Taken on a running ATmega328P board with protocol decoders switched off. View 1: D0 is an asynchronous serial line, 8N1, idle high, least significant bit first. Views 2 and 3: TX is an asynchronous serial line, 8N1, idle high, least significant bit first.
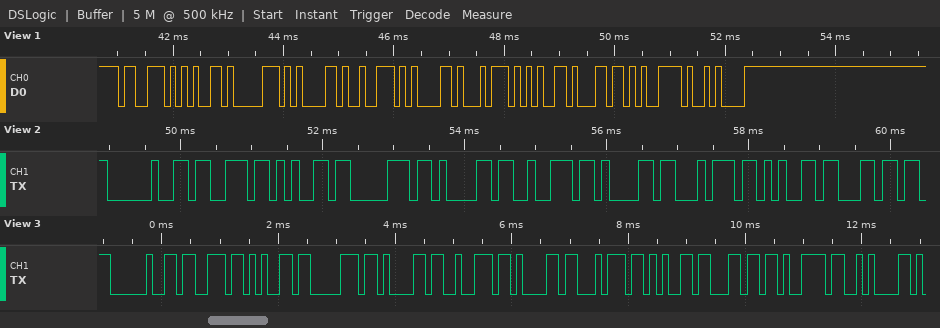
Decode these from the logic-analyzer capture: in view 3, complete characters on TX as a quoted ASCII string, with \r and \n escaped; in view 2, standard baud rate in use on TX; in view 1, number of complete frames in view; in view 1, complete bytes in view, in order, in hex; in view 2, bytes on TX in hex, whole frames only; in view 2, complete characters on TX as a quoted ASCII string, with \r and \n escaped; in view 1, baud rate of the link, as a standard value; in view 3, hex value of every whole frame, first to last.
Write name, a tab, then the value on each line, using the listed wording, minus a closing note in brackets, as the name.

in view 3, complete characters on TX as a quoted ASCII string, with \r and \n escaped	" separately\n"
in view 2, standard baud rate in use on TX	9600 baud
in view 1, number of complete frames in view	11
in view 1, complete bytes in view, in order, in hex	73 65 70 61 72 61 74 65 6C 79 0A
in view 2, bytes on TX in hex, whole frames only	20 73 65 70 61 72 61 74 65 6C
in view 2, complete characters on TX as a quoted ASCII string, with \r and \n escaped	" separatel"
in view 1, baud rate of the link, as a standard value	9600 baud
in view 3, hex value of every whole frame, first to last	20 73 65 70 61 72 61 74 65 6C 79 0A
